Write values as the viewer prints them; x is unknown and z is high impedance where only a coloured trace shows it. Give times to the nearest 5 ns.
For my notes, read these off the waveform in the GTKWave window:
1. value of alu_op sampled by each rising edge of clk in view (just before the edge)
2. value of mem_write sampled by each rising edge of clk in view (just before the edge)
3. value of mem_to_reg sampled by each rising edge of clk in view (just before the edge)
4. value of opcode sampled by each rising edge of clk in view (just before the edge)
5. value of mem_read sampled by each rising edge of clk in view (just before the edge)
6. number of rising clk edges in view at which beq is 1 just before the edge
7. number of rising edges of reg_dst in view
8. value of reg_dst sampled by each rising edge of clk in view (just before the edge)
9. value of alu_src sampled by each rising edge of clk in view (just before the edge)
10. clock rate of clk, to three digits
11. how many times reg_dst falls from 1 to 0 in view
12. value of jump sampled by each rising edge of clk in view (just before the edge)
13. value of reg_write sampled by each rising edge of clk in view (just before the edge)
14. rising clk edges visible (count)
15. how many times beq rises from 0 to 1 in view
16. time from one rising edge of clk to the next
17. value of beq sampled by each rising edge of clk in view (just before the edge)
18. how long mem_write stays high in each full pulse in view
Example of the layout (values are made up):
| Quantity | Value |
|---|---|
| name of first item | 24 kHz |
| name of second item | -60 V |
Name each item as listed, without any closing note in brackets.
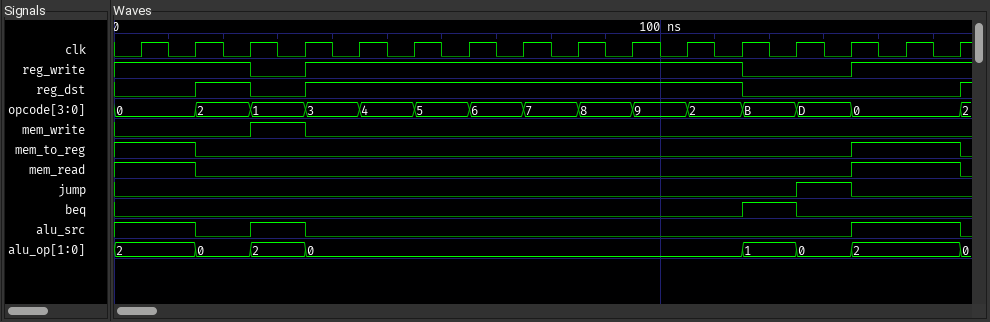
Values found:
| Quantity | Value |
|---|---|
| value of alu_op sampled by each rising edge of clk in view | 2, 2, 0, 2, 0, 0, 0, 0, 0, 0, 0, 0, 1, 0, 2, 2 |
| value of mem_write sampled by each rising edge of clk in view | 0 0 0 1 0 0 0 0 0 0 0 0 0 0 0 0 |
| value of mem_to_reg sampled by each rising edge of clk in view | 1 1 0 0 0 0 0 0 0 0 0 0 0 0 1 1 |
| value of opcode sampled by each rising edge of clk in view | 0, 0, 2, 1, 3, 4, 5, 6, 7, 8, 9, 2, B, D, 0, 0 |
| value of mem_read sampled by each rising edge of clk in view | 1 1 0 0 0 0 0 0 0 0 0 0 0 0 1 1 |
| number of rising clk edges in view at which beq is 1 just before the edge | 1 |
| number of rising edges of reg_dst in view | 3 |
| value of reg_dst sampled by each rising edge of clk in view | 0 0 1 0 1 1 1 1 1 1 1 1 0 0 0 0 |
| value of alu_src sampled by each rising edge of clk in view | 1 1 0 1 0 0 0 0 0 0 0 0 0 0 1 1 |
| clock rate of clk, to three digits | 100 MHz |
| how many times reg_dst falls from 1 to 0 in view | 2 |
| value of jump sampled by each rising edge of clk in view | 0 0 0 0 0 0 0 0 0 0 0 0 0 1 0 0 |
| value of reg_write sampled by each rising edge of clk in view | 1 1 1 0 1 1 1 1 1 1 1 1 0 0 1 1 |
| rising clk edges visible | 16 |
| how many times beq rises from 0 to 1 in view | 1 |
| time from one rising edge of clk to the next | 10 ns |
| value of beq sampled by each rising edge of clk in view | 0 0 0 0 0 0 0 0 0 0 0 0 1 0 0 0 |
| how long mem_write stays high in each full pulse in view | 10 ns |
